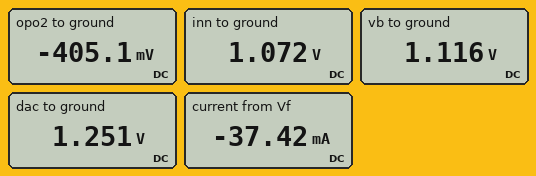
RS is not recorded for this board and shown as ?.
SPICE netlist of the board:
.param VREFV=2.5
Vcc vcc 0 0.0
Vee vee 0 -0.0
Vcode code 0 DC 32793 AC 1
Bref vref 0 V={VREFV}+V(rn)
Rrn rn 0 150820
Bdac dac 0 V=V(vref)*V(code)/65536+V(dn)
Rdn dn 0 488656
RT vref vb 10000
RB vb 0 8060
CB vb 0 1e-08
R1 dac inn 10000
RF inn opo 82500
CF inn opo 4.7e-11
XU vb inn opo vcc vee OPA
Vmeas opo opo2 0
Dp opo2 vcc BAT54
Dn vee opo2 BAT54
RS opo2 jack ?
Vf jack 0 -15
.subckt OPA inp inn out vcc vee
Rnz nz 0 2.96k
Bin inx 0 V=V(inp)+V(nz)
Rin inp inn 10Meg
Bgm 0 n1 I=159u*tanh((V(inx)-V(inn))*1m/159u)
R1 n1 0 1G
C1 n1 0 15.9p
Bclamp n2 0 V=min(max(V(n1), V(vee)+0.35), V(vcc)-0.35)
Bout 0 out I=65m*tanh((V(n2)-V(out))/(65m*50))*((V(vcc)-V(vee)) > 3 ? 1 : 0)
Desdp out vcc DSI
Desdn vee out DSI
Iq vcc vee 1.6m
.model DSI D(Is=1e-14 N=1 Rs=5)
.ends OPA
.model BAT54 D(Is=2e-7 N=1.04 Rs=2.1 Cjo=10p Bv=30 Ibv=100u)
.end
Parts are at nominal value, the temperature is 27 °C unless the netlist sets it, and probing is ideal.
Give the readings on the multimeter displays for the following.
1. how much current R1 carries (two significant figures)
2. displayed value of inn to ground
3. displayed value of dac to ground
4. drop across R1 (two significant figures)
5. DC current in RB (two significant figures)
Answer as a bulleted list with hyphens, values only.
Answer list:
- 18 µA
- 1.072 V
- 1.251 V
- 180 mV
- 140 µA
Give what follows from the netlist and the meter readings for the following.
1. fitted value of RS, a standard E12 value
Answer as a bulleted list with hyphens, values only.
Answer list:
- 390 Ω
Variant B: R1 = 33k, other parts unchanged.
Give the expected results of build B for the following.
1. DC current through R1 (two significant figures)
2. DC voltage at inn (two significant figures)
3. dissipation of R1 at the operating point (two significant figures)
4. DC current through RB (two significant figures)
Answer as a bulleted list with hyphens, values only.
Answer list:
- 14 µA
- 780 mV
- 6.8 µW
- 140 µA
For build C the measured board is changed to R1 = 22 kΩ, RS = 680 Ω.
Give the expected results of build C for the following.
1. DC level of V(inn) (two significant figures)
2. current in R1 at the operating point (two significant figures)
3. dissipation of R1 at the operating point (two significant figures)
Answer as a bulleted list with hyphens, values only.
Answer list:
- 910 mV
- 15 µA
- 5.2 µW
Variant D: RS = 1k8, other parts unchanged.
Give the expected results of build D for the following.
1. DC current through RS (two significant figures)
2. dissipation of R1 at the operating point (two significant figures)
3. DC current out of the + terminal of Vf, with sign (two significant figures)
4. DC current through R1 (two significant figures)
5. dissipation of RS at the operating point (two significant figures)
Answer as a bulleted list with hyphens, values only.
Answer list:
- 8.2 mA
- 2.8 µW
- -8.2 mA
- 17 µA
- 120 mW
